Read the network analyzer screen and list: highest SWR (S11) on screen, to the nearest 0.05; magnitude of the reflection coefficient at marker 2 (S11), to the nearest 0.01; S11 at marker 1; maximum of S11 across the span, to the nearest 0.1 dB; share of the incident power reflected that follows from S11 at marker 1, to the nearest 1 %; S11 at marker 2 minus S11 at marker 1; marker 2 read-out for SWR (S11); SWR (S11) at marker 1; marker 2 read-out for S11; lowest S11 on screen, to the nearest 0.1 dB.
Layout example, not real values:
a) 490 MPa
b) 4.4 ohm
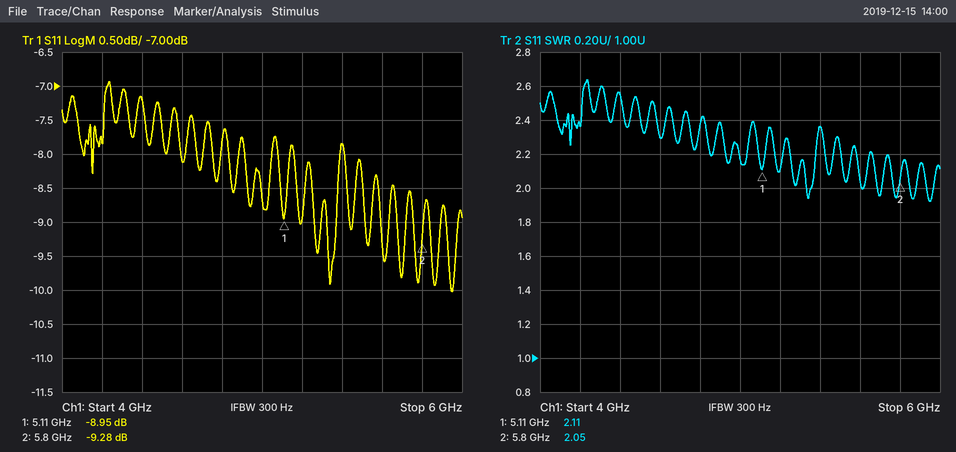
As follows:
a) 2.65
b) 0.34
c) -8.95 dB
d) -6.9 dB
e) 13 %
f) -0.33 dB
g) 2.05
h) 2.11
i) -9.28 dB
j) -10.0 dB
